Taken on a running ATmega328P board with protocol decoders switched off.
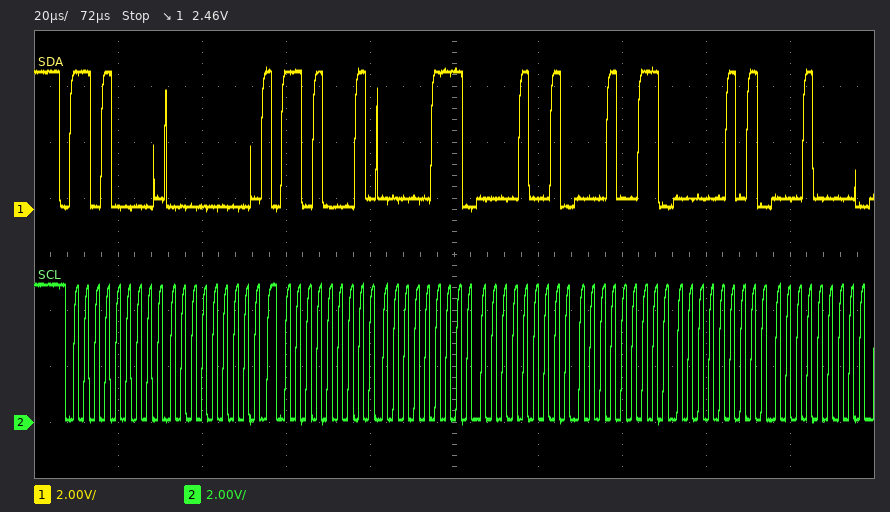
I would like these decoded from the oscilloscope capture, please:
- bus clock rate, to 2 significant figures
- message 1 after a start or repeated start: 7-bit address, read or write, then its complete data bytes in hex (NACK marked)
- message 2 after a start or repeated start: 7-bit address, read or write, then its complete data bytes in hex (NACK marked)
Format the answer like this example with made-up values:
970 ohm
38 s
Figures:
400 kHz
0x68 write: 00
0x68 read: 07 09 13 05 10
